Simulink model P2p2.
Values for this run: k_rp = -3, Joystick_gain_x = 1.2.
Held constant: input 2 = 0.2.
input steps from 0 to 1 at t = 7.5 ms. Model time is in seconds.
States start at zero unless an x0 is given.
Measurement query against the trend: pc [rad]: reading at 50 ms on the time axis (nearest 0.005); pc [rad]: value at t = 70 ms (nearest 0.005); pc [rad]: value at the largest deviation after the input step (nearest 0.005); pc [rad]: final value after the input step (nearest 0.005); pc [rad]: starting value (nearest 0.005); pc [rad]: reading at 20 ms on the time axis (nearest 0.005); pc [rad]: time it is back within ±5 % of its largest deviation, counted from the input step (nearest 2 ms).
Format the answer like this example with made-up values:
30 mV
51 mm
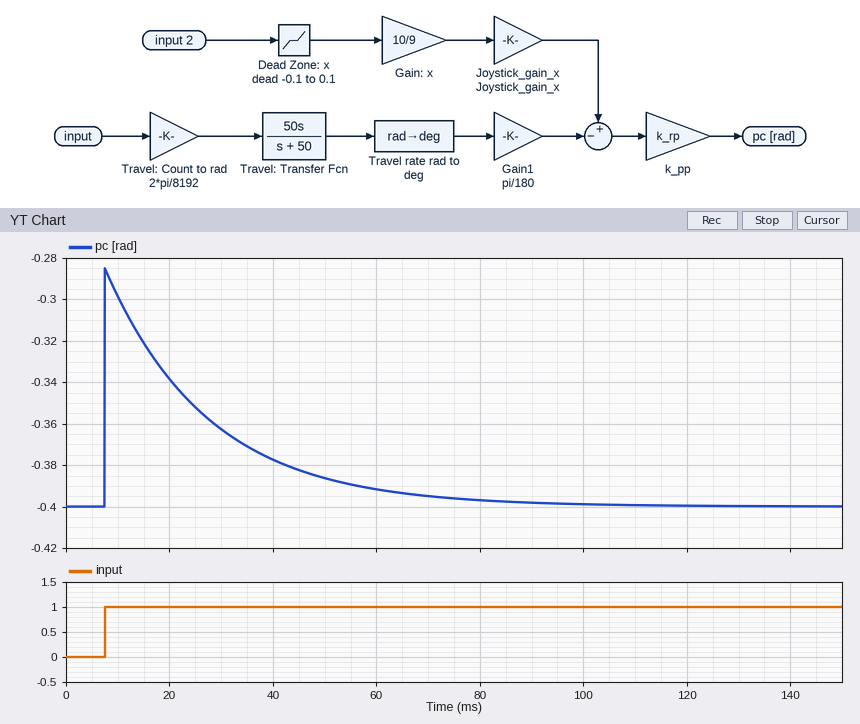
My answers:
-0.385
-0.395
-0.285
-0.400
-0.400
-0.340
60 ms
